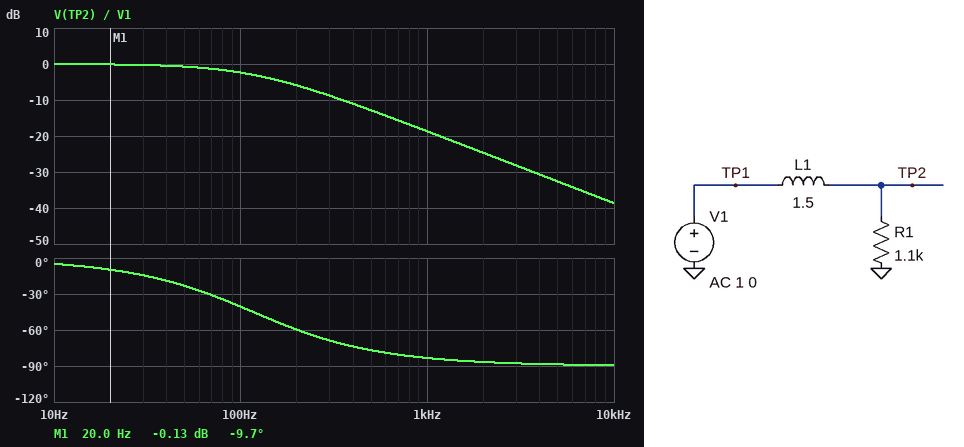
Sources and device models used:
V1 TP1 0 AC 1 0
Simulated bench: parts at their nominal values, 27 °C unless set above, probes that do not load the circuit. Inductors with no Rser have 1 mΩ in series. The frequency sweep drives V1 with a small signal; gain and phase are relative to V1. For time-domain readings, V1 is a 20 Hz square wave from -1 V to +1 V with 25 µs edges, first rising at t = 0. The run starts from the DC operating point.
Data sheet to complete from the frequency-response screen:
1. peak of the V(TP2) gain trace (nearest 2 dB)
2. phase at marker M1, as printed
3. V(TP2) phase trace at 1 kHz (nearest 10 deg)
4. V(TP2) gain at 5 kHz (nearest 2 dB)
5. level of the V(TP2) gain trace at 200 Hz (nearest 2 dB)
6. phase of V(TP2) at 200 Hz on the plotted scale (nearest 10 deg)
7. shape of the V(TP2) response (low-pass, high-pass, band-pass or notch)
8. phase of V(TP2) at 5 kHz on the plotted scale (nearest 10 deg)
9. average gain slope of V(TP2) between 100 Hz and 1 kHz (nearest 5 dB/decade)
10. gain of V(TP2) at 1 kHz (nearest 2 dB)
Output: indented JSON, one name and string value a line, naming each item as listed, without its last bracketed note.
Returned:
{
  "peak of the V(TP2) gain trace": "0 dB",
  "phase at marker M1, as printed": "-9.7 deg",
  "V(TP2) phase trace at 1 kHz": "-80 deg",
  "V(TP2) gain at 5 kHz": "-32 dB",
  "level of the V(TP2) gain trace at 200 Hz": "-6 dB",
  "phase of V(TP2) at 200 Hz on the plotted scale": "-60 deg",
  "shape of the V(TP2) response": "low-pass",
  "phase of V(TP2) at 5 kHz on the plotted scale": "-90 deg",
  "average gain slope of V(TP2) between 100 Hz and 1 kHz": "-15 dB/decade",
  "gain of V(TP2) at 1 kHz": "-18 dB"
}
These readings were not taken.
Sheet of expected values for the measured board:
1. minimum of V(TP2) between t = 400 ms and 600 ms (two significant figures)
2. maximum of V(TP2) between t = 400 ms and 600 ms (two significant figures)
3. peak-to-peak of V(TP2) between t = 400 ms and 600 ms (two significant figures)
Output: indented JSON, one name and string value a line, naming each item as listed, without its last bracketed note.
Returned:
{
  "minimum of V(TP2) between t = 400 ms and 600 ms": "-1.0 V",
  "maximum of V(TP2) between t = 400 ms and 600 ms": "1.0 V",
  "peak-to-peak of V(TP2) between t = 400 ms and 600 ms": "2.0 V"
}
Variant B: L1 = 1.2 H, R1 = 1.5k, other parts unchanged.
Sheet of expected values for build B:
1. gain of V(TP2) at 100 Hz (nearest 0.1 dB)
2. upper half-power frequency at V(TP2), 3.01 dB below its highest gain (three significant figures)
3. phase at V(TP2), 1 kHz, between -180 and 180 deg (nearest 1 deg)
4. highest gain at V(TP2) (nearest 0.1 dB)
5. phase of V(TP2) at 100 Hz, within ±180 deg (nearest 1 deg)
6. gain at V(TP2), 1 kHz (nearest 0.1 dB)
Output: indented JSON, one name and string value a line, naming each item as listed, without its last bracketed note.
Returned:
{
  "gain of V(TP2) at 100 Hz": "-1.0 dB",
  "upper half-power frequency at V(TP2), 3.01 dB below its highest gain": "199 Hz",
  "phase at V(TP2), 1 kHz, between -180 and 180 deg": "-79 deg",
  "highest gain at V(TP2)": "0 dB",
  "phase of V(TP2) at 100 Hz, within ±180 deg": "-27 deg",
  "gain at V(TP2), 1 kHz": "-14.2 dB"
}
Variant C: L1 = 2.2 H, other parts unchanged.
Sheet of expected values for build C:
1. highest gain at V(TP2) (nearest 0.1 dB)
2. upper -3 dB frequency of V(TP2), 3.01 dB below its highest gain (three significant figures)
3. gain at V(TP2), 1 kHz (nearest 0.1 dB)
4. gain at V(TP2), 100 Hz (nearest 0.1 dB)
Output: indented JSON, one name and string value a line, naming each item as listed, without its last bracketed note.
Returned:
{
  "highest gain at V(TP2)": "0 dB",
  "upper -3 dB frequency of V(TP2), 3.01 dB below its highest gain": "79.6 Hz",
  "gain at V(TP2), 1 kHz": "-22.0 dB",
  "gain at V(TP2), 100 Hz": "-4.1 dB"
}
